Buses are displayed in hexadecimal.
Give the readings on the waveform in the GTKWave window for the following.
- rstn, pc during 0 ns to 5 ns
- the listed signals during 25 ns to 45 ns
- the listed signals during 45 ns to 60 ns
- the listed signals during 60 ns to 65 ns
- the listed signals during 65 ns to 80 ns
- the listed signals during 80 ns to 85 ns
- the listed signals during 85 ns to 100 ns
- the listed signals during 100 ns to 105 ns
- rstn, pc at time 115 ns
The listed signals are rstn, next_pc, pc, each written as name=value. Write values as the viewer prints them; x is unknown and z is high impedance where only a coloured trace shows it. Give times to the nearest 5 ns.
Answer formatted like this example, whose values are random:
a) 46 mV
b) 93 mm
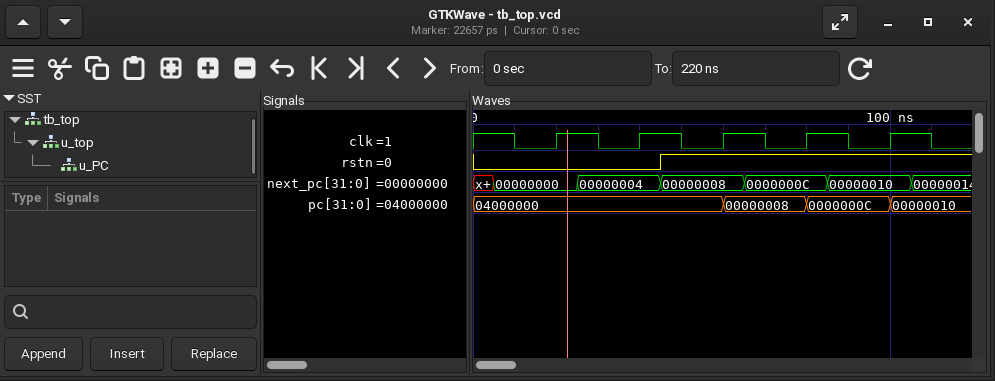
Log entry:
a) rstn=0, pc=04000000
b) rstn=0, next_pc=00000004, pc=04000000
c) rstn=1, next_pc=00000008, pc=04000000
d) rstn=1, next_pc=00000008, pc=00000008
e) rstn=1, next_pc=0000000C, pc=00000008
f) rstn=1, next_pc=0000000C, pc=0000000C
g) rstn=1, next_pc=00000010, pc=0000000C
h) rstn=1, next_pc=00000010, pc=00000010
i) rstn=1, pc=00000010
